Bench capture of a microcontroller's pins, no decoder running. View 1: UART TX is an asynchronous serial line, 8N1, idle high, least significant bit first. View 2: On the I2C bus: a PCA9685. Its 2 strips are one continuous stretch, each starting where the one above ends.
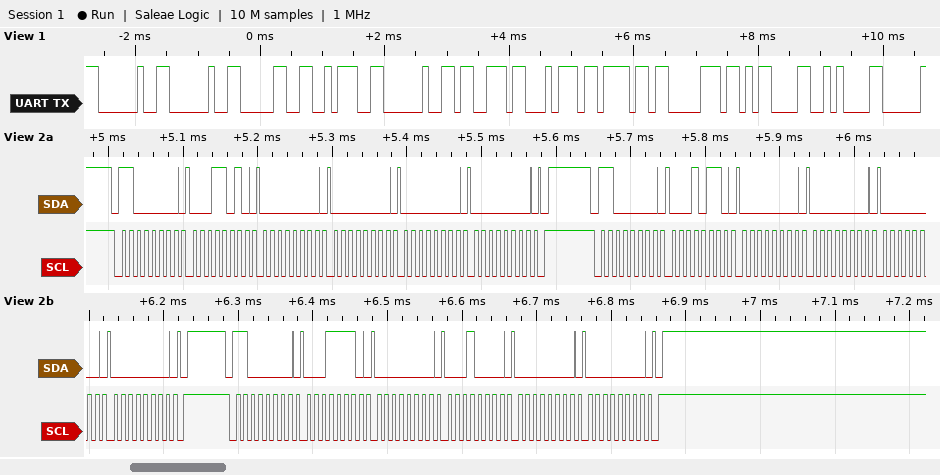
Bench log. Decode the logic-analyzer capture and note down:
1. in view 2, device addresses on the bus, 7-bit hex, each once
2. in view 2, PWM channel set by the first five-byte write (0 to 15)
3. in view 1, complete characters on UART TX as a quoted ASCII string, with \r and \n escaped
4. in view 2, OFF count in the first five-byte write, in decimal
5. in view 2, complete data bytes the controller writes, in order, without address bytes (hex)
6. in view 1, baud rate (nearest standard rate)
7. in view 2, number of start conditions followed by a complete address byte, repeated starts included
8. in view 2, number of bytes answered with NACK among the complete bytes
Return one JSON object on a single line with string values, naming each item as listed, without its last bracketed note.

{"in view 2, device addresses on the bus, 7-bit hex, each once": "0x60", "in view 2, PWM channel set by the first five-byte write": "5", "in view 1, complete characters on UART TX as a quoted ASCII string, with \\r and \\n escaped": "\"  0: stop\\r\\n\"", "in view 2, OFF count in the first five-byte write, in decimal": "0", "in view 2, complete data bytes the controller writes, in order, without address bytes": "1A 00 00 00 00 16 00 00 00 00 1E 00 10 00 00", "in view 1, baud rate": "9600 baud", "in view 2, number of start conditions followed by a complete address byte, repeated starts included": "3", "in view 2, number of bytes answered with NACK among the complete bytes": "0"}
